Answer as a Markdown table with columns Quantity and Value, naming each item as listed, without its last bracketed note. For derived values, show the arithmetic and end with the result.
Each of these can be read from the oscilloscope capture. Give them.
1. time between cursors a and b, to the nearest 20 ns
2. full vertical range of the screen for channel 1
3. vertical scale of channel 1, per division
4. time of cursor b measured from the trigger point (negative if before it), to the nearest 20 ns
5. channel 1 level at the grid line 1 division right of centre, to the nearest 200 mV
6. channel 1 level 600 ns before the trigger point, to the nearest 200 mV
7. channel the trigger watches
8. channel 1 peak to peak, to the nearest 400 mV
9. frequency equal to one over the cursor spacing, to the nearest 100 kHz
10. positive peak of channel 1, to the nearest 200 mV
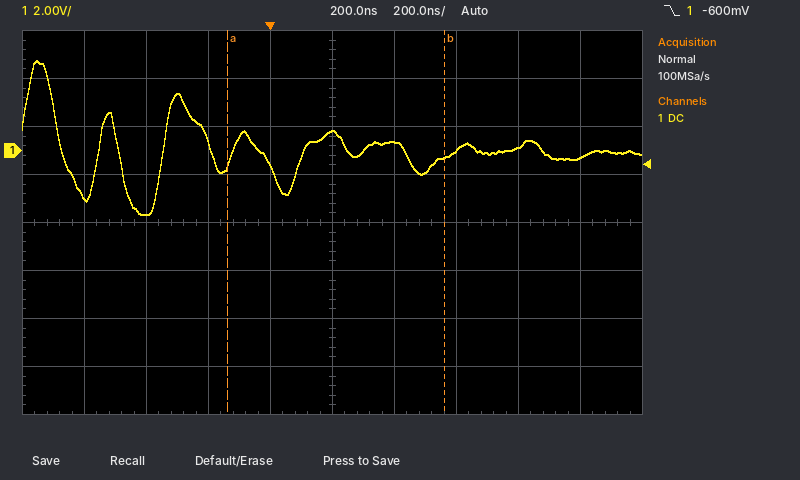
| Quantity | Value |
|---|---|
| time between cursors a and b, to the nearest 20 ns | 700 ns |
| full vertical range of the screen for channel 1 | 16 V |
| vertical scale of channel 1, per division | 2 V |
| time of cursor b measured from the trigger point (negative if before it), to the nearest 20 ns | +560 ns |
| channel 1 level at the grid line 1 division right of centre, to the nearest 200 mV | 400 mV |
| channel 1 level 600 ns before the trigger point, to the nearest 200 mV | -2.0 V |
| channel the trigger watches | channel 1 |
| channel 1 peak to peak, to the nearest 400 mV | 6.4 V |
| frequency equal to one over the cursor spacing, to the nearest 100 kHz | 1 / 700 ns ≈ 1.4 MHz |
| positive peak of channel 1, to the nearest 200 mV | 3.8 V |
